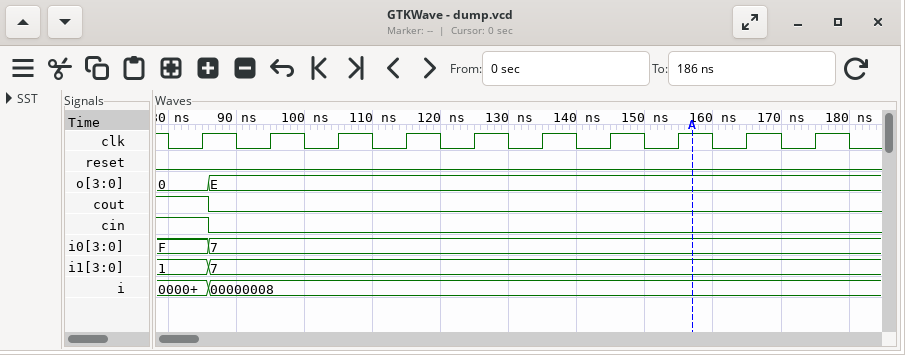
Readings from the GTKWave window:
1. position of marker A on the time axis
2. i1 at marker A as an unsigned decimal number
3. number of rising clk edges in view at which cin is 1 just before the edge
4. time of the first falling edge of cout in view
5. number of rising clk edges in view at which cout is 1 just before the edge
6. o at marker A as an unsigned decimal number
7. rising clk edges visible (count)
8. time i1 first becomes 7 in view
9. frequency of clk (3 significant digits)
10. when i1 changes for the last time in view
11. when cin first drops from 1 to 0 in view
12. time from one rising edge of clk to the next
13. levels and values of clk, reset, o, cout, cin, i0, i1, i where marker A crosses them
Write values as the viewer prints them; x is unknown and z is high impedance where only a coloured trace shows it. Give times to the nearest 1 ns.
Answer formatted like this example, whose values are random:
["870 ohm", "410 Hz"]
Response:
["157 ns", "7", "1", "86 ns", "1", "14", "10", "86 ns", "100 MHz", "86 ns", "86 ns", "10 ns", "clk=1, reset=0, o=E, cout=0, cin=0, i0=7, i1=7, i=00000008"]
